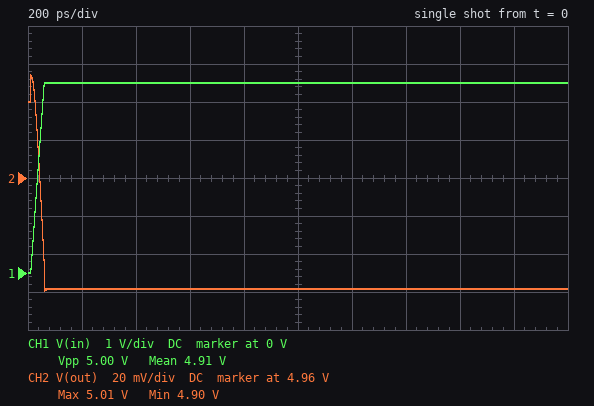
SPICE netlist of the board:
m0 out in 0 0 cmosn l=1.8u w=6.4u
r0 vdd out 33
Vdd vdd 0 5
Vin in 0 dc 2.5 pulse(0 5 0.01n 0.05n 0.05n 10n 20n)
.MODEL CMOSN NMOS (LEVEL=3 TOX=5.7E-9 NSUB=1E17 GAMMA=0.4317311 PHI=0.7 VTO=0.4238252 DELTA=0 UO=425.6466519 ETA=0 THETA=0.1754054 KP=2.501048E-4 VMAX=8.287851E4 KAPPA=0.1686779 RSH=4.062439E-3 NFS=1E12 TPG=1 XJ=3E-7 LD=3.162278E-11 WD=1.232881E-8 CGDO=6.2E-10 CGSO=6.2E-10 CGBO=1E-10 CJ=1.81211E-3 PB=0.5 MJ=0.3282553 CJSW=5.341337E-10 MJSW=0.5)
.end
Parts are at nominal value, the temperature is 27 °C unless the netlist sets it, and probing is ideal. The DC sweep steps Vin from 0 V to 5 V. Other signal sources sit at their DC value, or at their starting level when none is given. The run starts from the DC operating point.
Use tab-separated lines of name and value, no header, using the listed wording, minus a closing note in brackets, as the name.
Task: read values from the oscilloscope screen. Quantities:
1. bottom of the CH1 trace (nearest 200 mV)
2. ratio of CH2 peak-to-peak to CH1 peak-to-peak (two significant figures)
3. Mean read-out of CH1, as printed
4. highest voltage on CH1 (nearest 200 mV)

bottom of the CH1 trace	0 V
ratio of CH2 peak-to-peak to CH1 peak-to-peak	0.023
Mean read-out of CH1, as printed	4.91 V
highest voltage on CH1	5.0 V
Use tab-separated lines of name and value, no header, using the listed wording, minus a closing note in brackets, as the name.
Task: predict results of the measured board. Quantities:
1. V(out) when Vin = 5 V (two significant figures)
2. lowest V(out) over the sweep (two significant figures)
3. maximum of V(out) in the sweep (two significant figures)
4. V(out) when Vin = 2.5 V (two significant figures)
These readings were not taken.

V(out) when Vin = 5 V	4.9 V
lowest V(out) over the sweep	4.9 V
maximum of V(out) in the sweep	5.0 V
V(out) when Vin = 2.5 V	5.0 V
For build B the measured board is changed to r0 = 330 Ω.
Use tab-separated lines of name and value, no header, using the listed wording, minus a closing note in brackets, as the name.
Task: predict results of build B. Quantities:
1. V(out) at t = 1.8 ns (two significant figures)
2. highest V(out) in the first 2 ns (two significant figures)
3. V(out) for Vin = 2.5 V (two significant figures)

V(out) at t = 1.8 ns	4.0 V
highest V(out) in the first 2 ns	5.1 V
V(out) for Vin = 2.5 V	4.7 V
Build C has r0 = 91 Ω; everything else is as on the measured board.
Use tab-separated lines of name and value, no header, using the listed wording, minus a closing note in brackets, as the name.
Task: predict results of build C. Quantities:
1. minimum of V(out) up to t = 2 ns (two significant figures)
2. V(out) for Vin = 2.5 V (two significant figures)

minimum of V(out) up to t = 2 ns	4.7 V
V(out) for Vin = 2.5 V	4.9 V
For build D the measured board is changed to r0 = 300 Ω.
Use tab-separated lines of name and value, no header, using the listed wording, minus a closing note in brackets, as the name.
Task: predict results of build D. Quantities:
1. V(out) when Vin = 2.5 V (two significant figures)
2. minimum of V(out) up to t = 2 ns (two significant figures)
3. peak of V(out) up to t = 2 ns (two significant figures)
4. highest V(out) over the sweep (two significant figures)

V(out) when Vin = 2.5 V	4.7 V
minimum of V(out) up to t = 2 ns	4.1 V
peak of V(out) up to t = 2 ns	5.1 V
highest V(out) over the sweep	5.0 V
